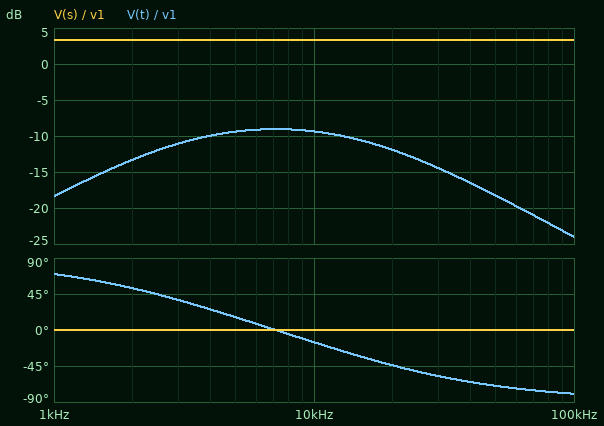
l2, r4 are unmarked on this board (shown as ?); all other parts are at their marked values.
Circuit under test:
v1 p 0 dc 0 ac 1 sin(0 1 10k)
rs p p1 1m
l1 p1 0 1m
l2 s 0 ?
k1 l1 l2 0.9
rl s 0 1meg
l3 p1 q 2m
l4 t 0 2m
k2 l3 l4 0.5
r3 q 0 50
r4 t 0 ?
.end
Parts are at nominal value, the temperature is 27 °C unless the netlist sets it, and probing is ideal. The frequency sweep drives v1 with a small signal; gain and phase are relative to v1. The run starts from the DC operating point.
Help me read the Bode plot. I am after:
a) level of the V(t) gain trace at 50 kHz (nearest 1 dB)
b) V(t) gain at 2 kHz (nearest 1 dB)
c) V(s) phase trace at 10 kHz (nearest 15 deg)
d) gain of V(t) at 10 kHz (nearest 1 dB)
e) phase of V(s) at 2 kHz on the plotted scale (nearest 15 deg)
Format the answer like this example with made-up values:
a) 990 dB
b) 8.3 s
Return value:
a) -18 dB
b) -13 dB
c) 0 deg
d) -9 dB
e) 0 deg
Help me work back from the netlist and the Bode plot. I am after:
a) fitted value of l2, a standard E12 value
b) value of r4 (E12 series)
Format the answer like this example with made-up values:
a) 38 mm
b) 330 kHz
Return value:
a) 2.7 mH
b) 120 Ω
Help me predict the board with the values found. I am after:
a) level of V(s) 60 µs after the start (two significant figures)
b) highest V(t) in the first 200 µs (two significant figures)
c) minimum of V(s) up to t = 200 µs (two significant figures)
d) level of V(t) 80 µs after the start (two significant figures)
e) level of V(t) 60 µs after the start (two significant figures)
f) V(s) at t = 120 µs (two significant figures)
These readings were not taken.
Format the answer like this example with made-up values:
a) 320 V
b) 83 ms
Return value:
a) -870 mV
b) 330 mV
c) -1.5 V
d) -370 mV
e) -170 mV
f) 1.4 V
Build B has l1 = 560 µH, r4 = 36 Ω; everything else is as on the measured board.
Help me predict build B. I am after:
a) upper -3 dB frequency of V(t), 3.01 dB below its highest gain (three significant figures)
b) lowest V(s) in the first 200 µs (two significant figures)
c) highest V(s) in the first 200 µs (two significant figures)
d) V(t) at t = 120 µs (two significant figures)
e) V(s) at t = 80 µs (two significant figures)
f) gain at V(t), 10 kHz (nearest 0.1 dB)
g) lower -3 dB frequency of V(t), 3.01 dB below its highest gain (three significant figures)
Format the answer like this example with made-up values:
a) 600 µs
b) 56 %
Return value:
a) 10.6 kHz
b) -2.0 V
c) 2.0 V
d) 59 mV
e) -1.9 V
f) -16.3 dB
g) 1.44 kHz
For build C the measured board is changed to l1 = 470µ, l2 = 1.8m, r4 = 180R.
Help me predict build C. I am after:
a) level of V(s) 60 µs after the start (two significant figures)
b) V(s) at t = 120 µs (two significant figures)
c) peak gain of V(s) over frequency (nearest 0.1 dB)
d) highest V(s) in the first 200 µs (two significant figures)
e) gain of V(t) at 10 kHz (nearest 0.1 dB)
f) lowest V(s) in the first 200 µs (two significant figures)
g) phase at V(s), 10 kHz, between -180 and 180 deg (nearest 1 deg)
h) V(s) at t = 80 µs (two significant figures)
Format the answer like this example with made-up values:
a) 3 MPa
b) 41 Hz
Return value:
a) -1.0 V
b) 1.7 V
c) 4.9 dB
d) 1.8 V
e) -8.2 dB
f) -1.8 V
g) 0 deg
h) -1.7 V
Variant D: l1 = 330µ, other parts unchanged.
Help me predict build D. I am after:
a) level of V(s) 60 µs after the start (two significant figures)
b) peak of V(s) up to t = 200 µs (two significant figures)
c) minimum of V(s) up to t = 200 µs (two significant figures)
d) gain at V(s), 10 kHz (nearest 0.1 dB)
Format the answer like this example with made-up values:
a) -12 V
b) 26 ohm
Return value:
a) -1.5 V
b) 2.6 V
c) -2.6 V
d) 8.2 dB
